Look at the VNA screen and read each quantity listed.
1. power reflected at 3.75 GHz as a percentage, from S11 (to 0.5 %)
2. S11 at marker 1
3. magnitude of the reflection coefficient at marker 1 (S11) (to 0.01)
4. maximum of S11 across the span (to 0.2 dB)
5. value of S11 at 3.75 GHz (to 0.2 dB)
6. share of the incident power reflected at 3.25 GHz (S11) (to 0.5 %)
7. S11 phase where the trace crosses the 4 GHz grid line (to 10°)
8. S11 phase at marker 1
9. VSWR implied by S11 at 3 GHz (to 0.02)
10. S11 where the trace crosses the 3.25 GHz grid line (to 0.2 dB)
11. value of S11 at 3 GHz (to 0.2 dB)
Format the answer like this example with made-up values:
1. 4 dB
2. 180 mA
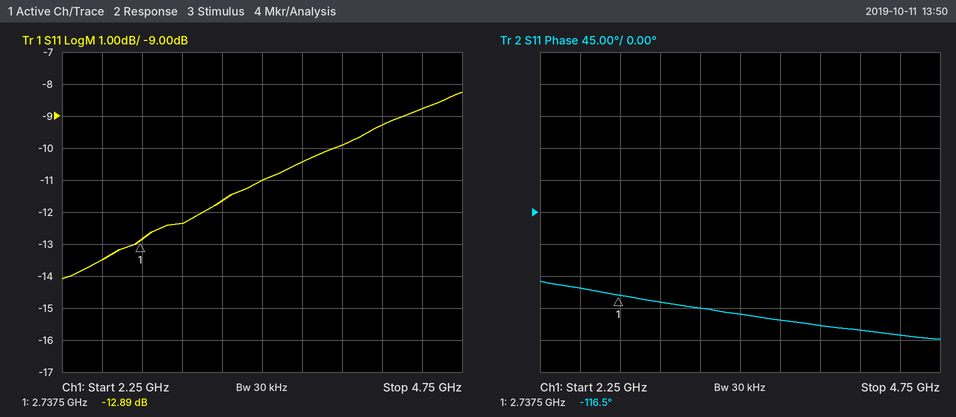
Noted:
1. 9.0 %
2. -12.89 dB
3. 0.23
4. -8.2 dB
5. -10.4 dB
6. 7.0 %
7. -160°
8. -116.5°
9. 1.64
10. -11.6 dB
11. -12.4 dB
